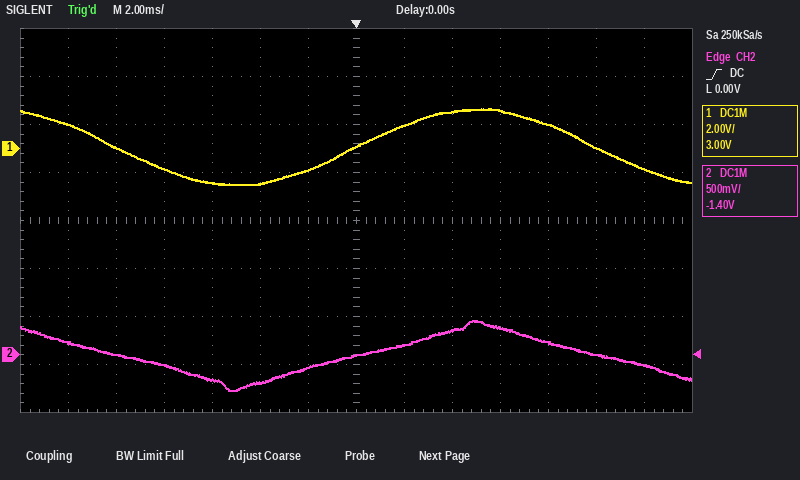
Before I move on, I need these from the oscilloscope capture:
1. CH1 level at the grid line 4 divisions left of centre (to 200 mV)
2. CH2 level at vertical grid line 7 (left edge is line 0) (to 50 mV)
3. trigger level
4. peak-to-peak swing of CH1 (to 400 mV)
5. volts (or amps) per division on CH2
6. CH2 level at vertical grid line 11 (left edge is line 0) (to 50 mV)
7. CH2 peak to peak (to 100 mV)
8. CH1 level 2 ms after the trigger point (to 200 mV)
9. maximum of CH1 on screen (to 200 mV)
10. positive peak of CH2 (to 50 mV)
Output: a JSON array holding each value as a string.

["-800 mV", "0 mV", "0.00 V", "3.2 V", "500 mV", "150 mV", "700 mV", "1.0 V", "1.6 V", "350 mV"]
